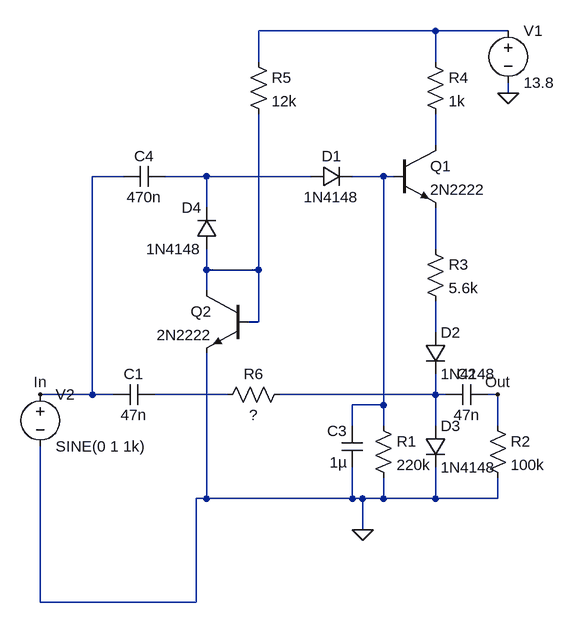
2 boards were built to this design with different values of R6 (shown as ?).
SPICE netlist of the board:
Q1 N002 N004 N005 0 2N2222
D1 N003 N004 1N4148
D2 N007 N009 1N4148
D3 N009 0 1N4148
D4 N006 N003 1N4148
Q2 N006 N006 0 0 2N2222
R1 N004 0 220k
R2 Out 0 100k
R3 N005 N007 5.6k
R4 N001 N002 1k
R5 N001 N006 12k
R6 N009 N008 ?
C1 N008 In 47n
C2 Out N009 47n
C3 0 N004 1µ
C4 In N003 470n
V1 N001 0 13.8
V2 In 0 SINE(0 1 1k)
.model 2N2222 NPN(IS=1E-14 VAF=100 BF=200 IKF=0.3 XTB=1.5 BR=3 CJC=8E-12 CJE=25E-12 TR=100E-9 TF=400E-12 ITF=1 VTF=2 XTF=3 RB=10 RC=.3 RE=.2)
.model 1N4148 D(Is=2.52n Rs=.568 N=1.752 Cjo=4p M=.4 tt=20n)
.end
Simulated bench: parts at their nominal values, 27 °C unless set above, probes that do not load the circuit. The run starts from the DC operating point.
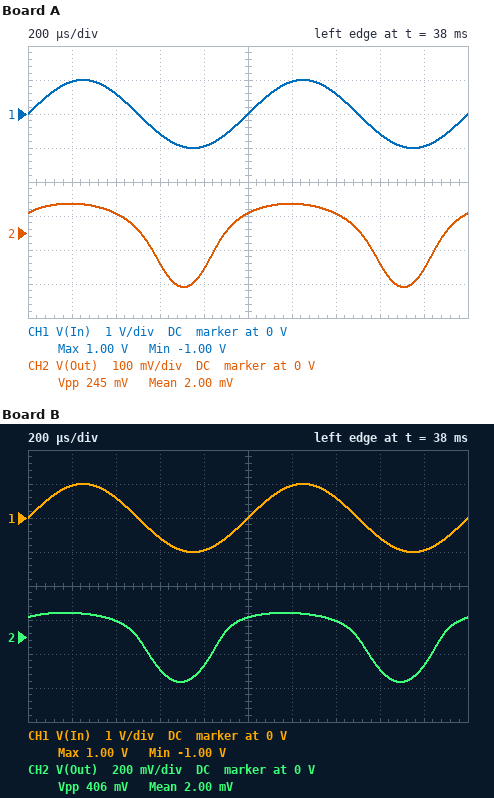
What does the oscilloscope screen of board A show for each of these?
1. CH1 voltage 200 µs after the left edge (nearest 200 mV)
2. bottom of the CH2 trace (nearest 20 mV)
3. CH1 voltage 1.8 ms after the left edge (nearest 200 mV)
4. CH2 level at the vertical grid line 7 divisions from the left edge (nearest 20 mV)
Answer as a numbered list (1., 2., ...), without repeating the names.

1. 1.0 V
2. -160 mV
3. -1.0 V
4. 60 mV
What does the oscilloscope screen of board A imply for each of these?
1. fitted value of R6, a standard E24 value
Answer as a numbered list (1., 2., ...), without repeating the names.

1. 11 kΩ
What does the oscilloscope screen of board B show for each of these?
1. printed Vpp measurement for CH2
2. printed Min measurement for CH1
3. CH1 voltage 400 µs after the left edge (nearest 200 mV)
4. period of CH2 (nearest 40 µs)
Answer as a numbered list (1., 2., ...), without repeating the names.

1. 406 mV
2. -1.00 V
3. 600 mV
4. 1.00 ms
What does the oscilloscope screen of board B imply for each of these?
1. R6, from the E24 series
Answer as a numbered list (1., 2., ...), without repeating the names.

1. 6.8 kΩ
